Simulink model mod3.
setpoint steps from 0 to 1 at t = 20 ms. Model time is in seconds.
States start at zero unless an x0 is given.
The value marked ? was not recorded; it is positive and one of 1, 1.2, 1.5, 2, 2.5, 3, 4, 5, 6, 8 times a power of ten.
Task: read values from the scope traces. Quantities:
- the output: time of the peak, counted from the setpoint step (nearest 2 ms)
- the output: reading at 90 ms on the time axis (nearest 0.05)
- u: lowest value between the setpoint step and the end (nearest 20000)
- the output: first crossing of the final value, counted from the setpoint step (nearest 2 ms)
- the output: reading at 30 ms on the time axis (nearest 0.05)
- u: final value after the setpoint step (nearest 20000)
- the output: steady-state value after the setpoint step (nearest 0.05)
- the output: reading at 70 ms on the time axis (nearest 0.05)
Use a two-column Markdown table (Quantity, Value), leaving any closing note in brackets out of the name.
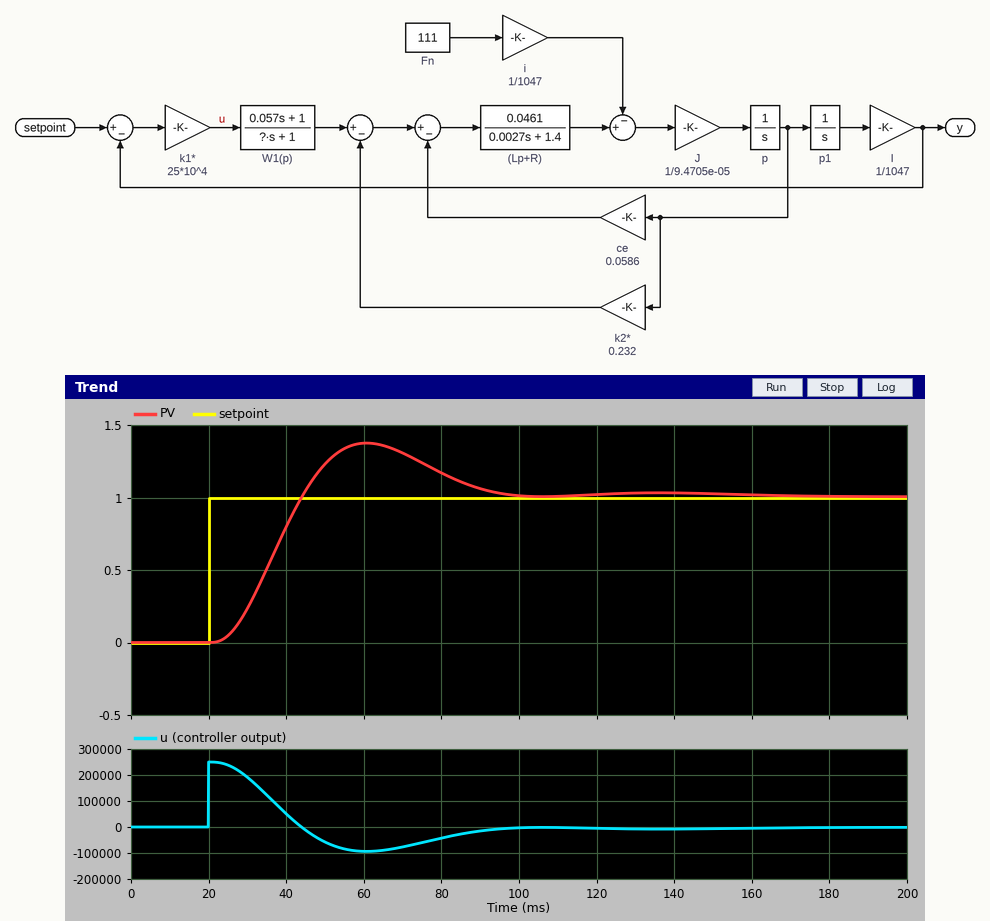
| Quantity | Value |
|---|---|
| the output: time of the peak, counted from the setpoint step | 40 ms |
| the output: reading at 90 ms on the time axis | 1.05 |
| u: lowest value between the setpoint step and the end | -100000 |
| the output: first crossing of the final value, counted from the setpoint step | 24 ms |
| the output: reading at 30 ms on the time axis | 0.25 |
| u: final value after the setpoint step | 0 |
| the output: steady-state value after the setpoint step | 1.00 |
| the output: reading at 70 ms on the time axis | 1.30 |
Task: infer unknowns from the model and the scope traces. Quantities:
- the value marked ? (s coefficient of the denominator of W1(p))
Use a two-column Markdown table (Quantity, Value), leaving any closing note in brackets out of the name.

| Quantity | Value |
|---|---|
| the value marked ? (s coefficient of the denominator of W1(p)) | 0.6 |
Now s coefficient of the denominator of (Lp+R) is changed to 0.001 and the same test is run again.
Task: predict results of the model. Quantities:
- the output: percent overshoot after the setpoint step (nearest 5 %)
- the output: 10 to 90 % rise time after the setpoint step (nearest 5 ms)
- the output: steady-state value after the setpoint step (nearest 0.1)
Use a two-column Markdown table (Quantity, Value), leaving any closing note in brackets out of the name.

| Quantity | Value |
|---|---|
| the output: percent overshoot after the setpoint step | 35 % |
| the output: 10 to 90 % rise time after the setpoint step | 15 ms |
| the output: steady-state value after the setpoint step | 1.0 |
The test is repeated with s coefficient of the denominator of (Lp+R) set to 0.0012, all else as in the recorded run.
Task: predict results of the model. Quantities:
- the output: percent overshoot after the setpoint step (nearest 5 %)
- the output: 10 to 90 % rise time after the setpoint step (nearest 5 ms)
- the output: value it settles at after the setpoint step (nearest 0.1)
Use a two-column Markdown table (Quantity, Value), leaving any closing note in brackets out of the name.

| Quantity | Value |
|---|---|
| the output: percent overshoot after the setpoint step | 35 % |
| the output: 10 to 90 % rise time after the setpoint step | 15 ms |
| the output: value it settles at after the setpoint step | 1.0 |
